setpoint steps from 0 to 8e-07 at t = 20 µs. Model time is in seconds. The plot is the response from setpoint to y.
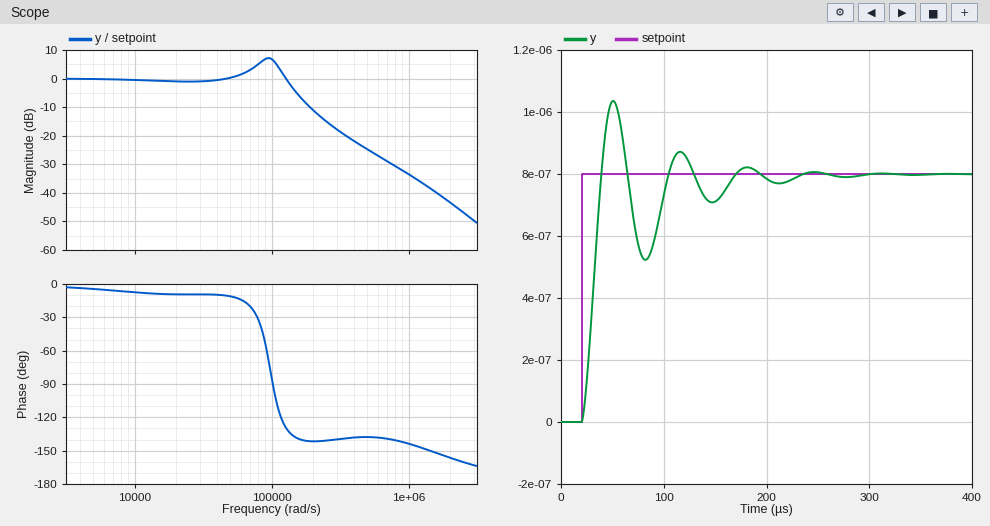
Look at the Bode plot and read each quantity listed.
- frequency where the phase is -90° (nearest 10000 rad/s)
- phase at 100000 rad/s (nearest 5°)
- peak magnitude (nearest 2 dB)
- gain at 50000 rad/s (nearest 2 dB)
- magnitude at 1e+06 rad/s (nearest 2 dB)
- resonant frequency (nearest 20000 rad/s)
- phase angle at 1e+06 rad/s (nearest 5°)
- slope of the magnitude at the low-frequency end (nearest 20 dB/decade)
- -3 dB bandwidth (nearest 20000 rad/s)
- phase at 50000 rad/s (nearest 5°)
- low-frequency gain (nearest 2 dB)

100000 rad/s
-85°
8 dB
0 dB
-34 dB
100000 rad/s
-145°
0 dB/decade
140000 rad/s
-10°
0 dB
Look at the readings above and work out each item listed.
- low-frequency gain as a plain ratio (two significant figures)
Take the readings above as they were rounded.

1.0
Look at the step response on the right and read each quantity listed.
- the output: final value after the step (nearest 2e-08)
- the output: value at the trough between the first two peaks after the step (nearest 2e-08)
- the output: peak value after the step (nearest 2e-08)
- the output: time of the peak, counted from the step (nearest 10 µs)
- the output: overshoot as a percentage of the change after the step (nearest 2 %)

0.00000080
0.00000052
0.00000104
30 µs
30 %
